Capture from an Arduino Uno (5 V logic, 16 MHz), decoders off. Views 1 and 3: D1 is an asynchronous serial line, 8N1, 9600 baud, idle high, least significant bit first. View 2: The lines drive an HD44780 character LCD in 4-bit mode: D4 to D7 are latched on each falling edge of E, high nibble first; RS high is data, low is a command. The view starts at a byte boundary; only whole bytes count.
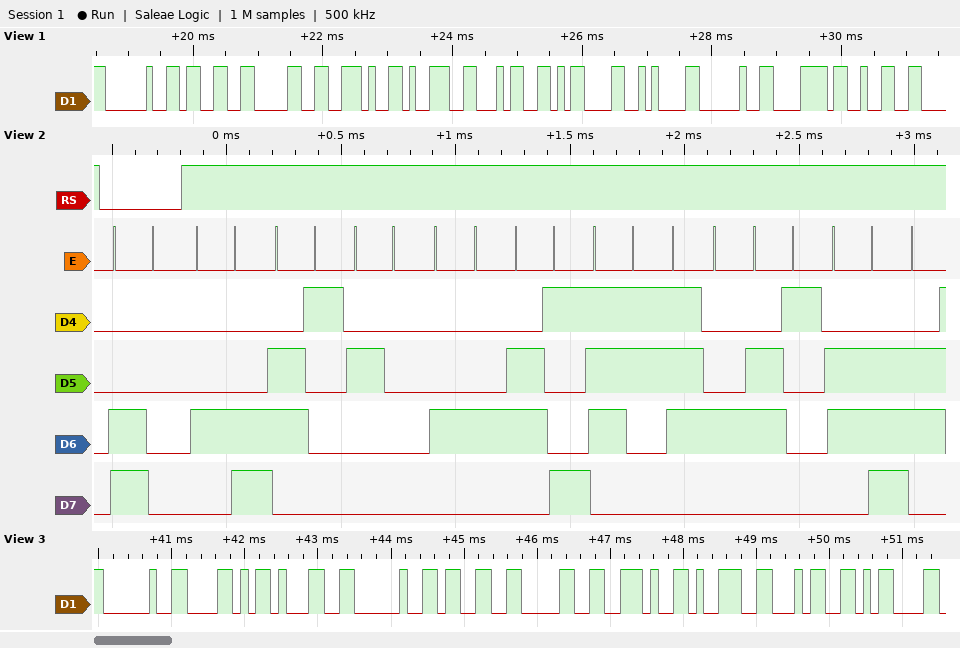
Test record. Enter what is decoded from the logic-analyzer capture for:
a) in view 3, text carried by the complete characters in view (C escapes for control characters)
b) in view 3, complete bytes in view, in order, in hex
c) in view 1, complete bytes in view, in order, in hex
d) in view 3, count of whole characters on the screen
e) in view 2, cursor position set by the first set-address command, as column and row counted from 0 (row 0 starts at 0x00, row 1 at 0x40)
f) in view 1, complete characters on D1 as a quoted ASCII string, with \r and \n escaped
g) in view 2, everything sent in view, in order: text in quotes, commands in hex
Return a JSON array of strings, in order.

["\" X1 30.94\\r\"", "20 58 31 20 33 30 2E 39 34 0D", "20 33 30 2E 39 34 0D 0A 20 78 32", "10", "column 0, row 1", "\" 30.94\\r\\n x2\"", "0xC0 \"La Distan\""]
